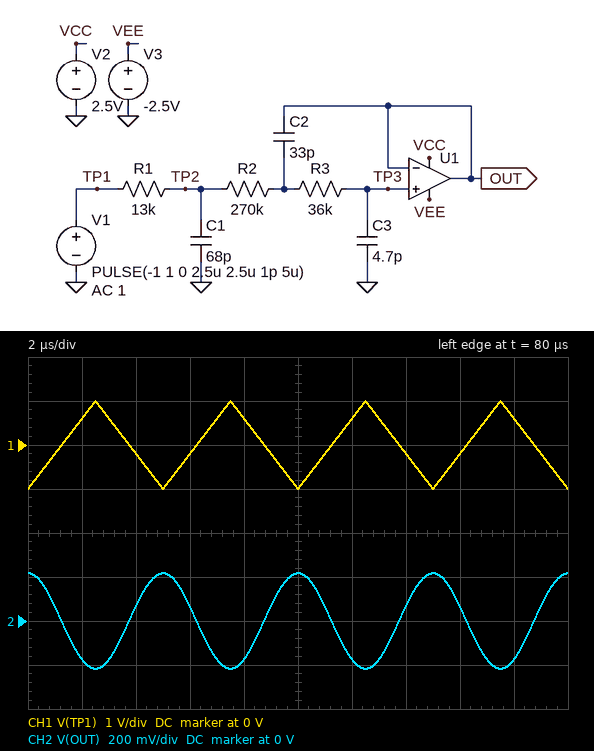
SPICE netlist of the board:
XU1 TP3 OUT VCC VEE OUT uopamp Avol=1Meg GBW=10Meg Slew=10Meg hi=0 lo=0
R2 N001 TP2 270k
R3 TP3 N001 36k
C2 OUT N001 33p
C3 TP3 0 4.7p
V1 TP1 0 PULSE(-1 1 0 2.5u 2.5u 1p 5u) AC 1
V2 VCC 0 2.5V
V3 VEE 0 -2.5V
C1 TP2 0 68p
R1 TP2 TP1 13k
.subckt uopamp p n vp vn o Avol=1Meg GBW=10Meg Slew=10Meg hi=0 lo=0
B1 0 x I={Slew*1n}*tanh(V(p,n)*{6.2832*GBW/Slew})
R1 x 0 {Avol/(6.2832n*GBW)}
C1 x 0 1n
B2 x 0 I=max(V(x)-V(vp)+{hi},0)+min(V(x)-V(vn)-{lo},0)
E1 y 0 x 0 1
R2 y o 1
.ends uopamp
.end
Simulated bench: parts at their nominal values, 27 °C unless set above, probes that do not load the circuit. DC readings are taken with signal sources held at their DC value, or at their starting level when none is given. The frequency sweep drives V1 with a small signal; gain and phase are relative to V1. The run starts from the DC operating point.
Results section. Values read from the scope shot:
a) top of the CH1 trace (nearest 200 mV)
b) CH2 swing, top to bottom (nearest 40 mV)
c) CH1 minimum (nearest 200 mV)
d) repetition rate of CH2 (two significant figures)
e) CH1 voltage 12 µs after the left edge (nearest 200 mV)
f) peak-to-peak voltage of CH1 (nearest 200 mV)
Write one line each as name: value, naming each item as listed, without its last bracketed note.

top of the CH1 trace: 1.0 V
CH2 swing, top to bottom: 440 mV
CH1 minimum: -1.0 V
repetition rate of CH2: 200 kHz
CH1 voltage 12 µs after the left edge: 600 mV
peak-to-peak voltage of CH1: 2.0 V
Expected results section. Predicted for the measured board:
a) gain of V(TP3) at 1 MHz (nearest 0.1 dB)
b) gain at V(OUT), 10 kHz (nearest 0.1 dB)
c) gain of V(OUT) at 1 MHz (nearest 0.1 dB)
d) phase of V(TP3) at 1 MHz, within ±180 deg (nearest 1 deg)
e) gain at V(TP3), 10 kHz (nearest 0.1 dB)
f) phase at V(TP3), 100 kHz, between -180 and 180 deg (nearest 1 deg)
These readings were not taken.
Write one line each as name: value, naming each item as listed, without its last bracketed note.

gain of V(TP3) at 1 MHz: -51.3 dB
gain at V(OUT), 10 kHz: 0 dB
gain of V(OUT) at 1 MHz: -51.3 dB
phase of V(TP3) at 1 MHz, within ±180 deg: 109 deg
gain at V(TP3), 10 kHz: 0 dB
phase at V(TP3), 100 kHz, between -180 and 180 deg: -99 deg
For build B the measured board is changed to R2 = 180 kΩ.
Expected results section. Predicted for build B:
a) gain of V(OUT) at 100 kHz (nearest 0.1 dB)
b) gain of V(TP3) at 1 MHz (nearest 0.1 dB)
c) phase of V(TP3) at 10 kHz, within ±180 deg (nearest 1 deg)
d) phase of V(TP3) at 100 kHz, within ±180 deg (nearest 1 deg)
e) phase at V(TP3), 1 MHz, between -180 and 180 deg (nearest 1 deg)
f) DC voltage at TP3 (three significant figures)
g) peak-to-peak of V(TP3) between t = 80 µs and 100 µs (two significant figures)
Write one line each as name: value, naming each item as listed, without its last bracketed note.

gain of V(OUT) at 100 kHz: -0.1 dB
gain of V(TP3) at 1 MHz: -47.7 dB
phase of V(TP3) at 10 kHz, within ±180 deg: -7 deg
phase of V(TP3) at 100 kHz, within ±180 deg: -80 deg
phase at V(TP3), 1 MHz, between -180 and 180 deg: 110 deg
DC voltage at TP3: -1.00 V
peak-to-peak of V(TP3) between t = 80 µs and 100 µs: 690 mV
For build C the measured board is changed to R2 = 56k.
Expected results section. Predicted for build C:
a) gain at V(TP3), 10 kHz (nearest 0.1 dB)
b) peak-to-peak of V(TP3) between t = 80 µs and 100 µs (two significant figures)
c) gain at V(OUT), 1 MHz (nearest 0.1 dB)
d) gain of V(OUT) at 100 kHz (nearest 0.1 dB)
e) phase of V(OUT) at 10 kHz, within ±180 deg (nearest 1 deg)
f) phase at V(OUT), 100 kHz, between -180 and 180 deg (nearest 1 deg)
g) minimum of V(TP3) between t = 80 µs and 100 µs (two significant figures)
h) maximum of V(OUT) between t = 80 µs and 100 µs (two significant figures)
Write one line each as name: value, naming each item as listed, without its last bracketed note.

gain at V(TP3), 10 kHz: 0 dB
peak-to-peak of V(TP3) between t = 80 µs and 100 µs: 1.4 V
gain at V(OUT), 1 MHz: -37.3 dB
gain of V(OUT) at 100 kHz: -0.4 dB
phase of V(OUT) at 10 kHz, within ±180 deg: -5 deg
phase at V(OUT), 100 kHz, between -180 and 180 deg: -50 deg
minimum of V(TP3) between t = 80 µs and 100 µs: -700 mV
maximum of V(OUT) between t = 80 µs and 100 µs: 700 mV
